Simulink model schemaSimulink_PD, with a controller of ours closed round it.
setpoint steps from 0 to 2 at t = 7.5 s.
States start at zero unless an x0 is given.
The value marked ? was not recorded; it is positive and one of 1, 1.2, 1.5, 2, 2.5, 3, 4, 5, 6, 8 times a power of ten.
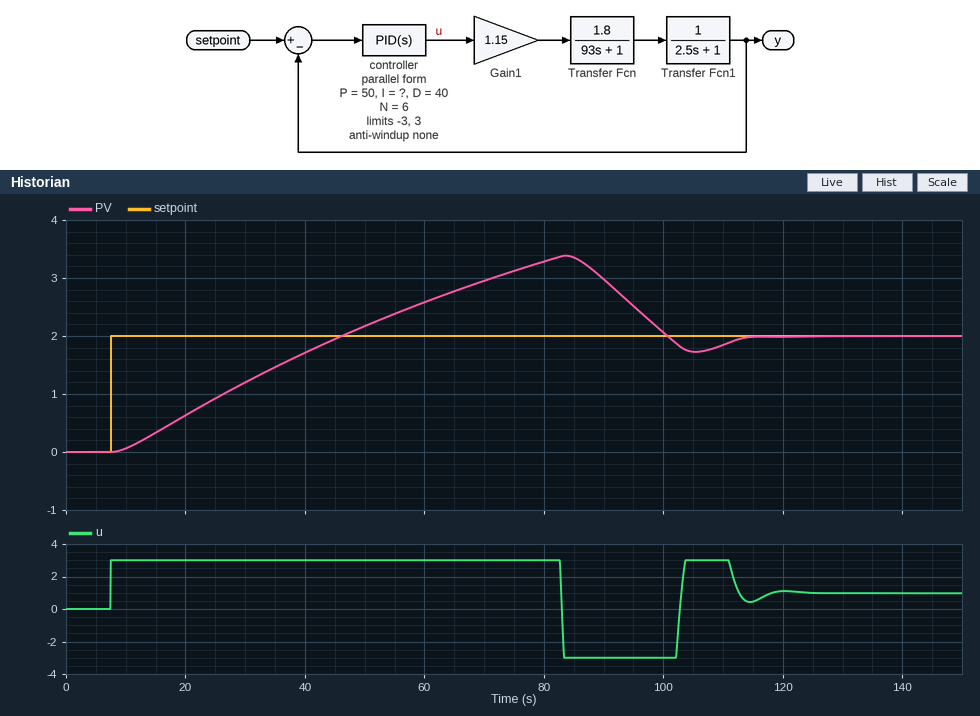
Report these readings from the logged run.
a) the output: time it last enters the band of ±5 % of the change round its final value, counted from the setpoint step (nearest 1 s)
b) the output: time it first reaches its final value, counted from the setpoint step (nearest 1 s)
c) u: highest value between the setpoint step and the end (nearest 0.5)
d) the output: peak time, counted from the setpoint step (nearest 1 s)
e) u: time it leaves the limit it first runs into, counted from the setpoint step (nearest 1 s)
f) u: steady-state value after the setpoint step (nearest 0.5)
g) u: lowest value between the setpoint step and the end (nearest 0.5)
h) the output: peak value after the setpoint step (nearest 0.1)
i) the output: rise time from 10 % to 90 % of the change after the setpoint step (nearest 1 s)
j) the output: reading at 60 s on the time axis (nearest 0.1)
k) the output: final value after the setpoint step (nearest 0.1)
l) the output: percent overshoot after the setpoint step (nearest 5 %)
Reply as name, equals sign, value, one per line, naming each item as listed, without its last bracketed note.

the output: time it last enters the band of ±5 % of the change round its final value, counted from the setpoint step = 104 s
the output: time it first reaches its final value, counted from the setpoint step = 39 s
u: highest value between the setpoint step and the end = 3.0
the output: peak time, counted from the setpoint step = 76 s
u: time it leaves the limit it first runs into, counted from the setpoint step = 75 s
u: steady-state value after the setpoint step = 1.0
u: lowest value between the setpoint step and the end = -3.0
the output: peak value after the setpoint step = 3.4
the output: rise time from 10 % to 90 % of the change after the setpoint step = 29 s
the output: reading at 60 s on the time axis = 2.6
the output: final value after the setpoint step = 2.0
the output: percent overshoot after the setpoint step = 70 %
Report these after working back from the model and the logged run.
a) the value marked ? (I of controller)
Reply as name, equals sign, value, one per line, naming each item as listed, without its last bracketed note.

the value marked ? = 6
